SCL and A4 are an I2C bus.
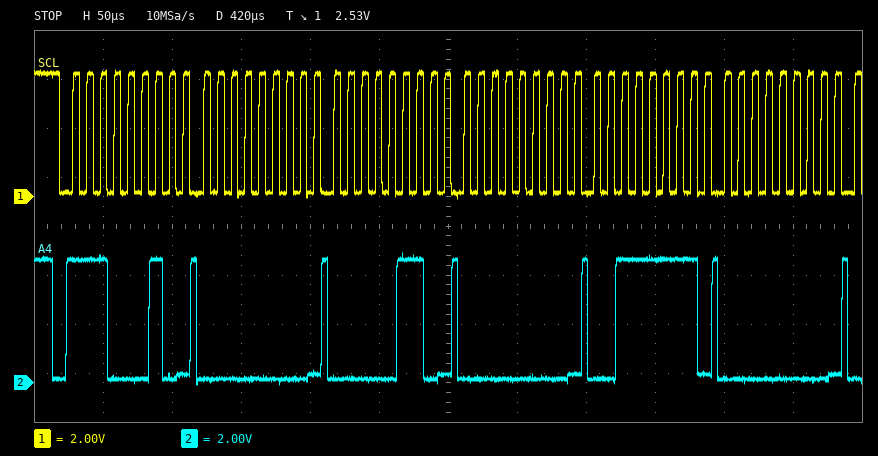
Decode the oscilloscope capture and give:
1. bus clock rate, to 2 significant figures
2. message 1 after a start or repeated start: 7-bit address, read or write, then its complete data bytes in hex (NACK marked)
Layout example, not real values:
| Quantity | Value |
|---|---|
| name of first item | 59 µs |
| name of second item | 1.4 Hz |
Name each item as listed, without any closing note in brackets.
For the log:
| Quantity | Value |
|---|---|
| bus clock rate, to 2 significant figures | 100 kHz |
| message 1 after a start or repeated start: 7-bit address, read or write, then its complete data bytes in hex | 0x71 write: 00 06 00 3F 00 |
